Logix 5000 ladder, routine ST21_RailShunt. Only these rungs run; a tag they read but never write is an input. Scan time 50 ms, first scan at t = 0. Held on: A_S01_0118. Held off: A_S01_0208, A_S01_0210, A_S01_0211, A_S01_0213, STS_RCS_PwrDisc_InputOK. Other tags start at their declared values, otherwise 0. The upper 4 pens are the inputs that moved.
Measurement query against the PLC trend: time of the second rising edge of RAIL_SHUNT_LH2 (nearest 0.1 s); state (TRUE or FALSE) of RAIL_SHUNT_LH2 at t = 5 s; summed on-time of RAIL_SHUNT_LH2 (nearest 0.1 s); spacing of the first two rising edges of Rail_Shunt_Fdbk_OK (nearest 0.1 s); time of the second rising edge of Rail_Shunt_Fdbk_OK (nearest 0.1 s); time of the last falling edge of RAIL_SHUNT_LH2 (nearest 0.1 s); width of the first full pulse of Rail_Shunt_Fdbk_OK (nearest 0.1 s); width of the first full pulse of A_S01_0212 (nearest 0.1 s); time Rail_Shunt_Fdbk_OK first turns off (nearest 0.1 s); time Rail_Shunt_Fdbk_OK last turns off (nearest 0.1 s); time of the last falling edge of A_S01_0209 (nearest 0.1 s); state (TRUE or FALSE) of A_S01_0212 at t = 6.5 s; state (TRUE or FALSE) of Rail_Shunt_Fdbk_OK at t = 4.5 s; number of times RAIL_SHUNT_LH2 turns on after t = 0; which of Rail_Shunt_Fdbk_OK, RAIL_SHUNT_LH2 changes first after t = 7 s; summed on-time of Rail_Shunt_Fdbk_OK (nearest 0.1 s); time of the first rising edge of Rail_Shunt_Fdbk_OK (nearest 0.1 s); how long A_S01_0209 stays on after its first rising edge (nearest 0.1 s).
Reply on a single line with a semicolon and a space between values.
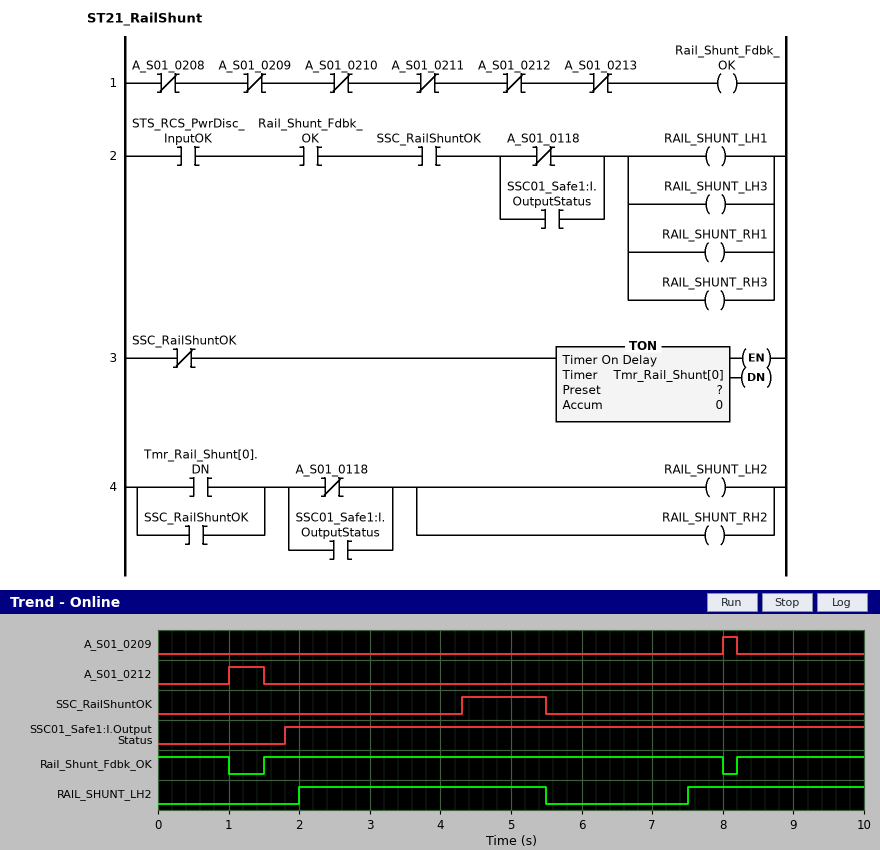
7.5 s; TRUE; 6.0 s; 6.7 s; 8.2 s; 5.5 s; 6.5 s; 0.5 s; 1.0 s; 8.0 s; 8.2 s; FALSE; TRUE; 2; RAIL_SHUNT_LH2; 9.3 s; 1.5 s; 0.2 s
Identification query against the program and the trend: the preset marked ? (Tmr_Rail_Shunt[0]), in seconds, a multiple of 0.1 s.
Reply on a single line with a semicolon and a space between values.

2.0 s
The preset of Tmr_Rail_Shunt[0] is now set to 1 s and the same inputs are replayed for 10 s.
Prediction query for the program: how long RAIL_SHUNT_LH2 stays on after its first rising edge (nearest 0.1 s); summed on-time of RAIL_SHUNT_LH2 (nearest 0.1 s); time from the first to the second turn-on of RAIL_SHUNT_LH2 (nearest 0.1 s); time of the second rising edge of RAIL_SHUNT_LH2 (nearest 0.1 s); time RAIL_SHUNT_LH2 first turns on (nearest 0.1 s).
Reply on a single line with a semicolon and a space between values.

3.7 s; 7.2 s; 4.7 s; 6.5 s; 1.8 s
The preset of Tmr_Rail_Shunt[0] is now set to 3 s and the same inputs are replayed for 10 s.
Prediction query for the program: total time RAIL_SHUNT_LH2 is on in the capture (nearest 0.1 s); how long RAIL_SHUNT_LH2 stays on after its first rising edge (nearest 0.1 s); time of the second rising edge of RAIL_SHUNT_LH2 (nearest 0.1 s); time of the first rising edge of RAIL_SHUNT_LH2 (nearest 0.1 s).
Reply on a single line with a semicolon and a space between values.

4.0 s; 2.5 s; 8.5 s; 3.0 s
